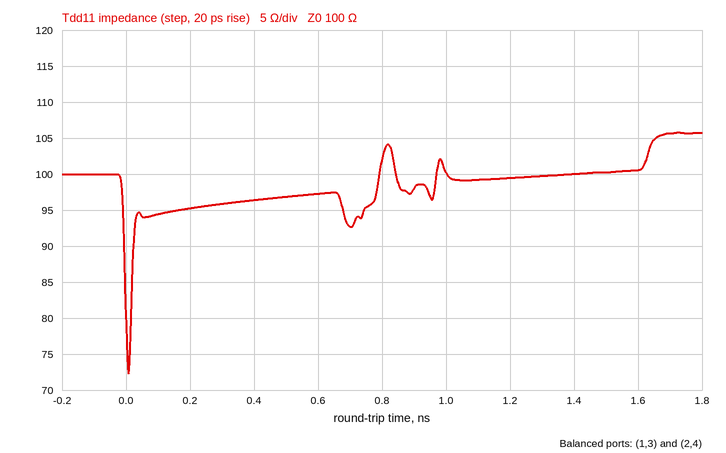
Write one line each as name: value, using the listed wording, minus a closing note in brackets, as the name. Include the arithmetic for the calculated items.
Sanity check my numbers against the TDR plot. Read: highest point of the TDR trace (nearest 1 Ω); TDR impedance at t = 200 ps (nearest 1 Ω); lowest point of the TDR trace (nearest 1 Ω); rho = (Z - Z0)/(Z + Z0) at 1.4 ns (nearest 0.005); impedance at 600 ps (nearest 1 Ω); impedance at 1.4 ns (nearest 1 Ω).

highest point of the TDR trace: 106 Ω
TDR impedance at t = 200 ps: 95 Ω
lowest point of the TDR trace: 72 Ω
rho = (Z - Z0)/(Z + Z0) at 1.4 ns: (100 − 100)/(100 + 100) ≈ 0.000
impedance at 600 ps: 97 Ω
impedance at 1.4 ns: 100 Ω
